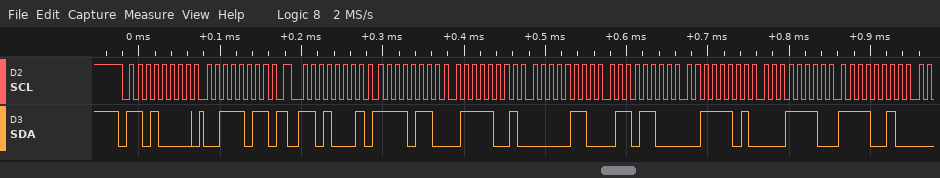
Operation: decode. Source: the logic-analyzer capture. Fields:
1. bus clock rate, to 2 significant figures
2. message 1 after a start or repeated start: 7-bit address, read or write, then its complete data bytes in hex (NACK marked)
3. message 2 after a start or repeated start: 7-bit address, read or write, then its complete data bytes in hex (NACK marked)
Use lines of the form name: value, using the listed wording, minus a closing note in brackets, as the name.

bus clock rate, to 2 significant figures: 100 kHz
message 1 after a start or repeated start: 7-bit address, read or write, then its complete data bytes in hex: 0x68 write: 3B
message 2 after a start or repeated start: 7-bit address, read or write, then its complete data bytes in hex: 0x68 read: F6 79 06 6C 3D 1E F2
